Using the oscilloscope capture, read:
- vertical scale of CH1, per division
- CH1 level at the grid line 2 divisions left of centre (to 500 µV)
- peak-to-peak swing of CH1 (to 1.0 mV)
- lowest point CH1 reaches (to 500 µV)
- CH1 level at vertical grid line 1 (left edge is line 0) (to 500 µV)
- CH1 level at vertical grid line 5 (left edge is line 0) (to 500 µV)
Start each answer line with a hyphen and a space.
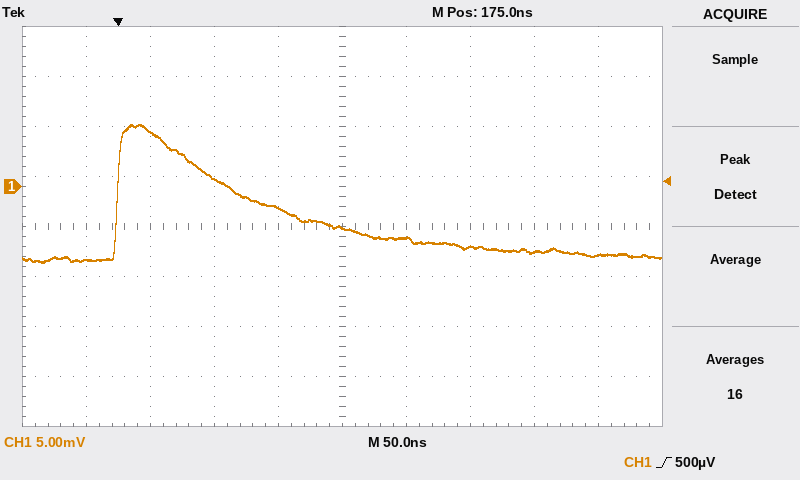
- 5 mV
- 1.0 mV
- 14.0 mV
- -7.5 mV
- -7.5 mV
- -4.0 mV
